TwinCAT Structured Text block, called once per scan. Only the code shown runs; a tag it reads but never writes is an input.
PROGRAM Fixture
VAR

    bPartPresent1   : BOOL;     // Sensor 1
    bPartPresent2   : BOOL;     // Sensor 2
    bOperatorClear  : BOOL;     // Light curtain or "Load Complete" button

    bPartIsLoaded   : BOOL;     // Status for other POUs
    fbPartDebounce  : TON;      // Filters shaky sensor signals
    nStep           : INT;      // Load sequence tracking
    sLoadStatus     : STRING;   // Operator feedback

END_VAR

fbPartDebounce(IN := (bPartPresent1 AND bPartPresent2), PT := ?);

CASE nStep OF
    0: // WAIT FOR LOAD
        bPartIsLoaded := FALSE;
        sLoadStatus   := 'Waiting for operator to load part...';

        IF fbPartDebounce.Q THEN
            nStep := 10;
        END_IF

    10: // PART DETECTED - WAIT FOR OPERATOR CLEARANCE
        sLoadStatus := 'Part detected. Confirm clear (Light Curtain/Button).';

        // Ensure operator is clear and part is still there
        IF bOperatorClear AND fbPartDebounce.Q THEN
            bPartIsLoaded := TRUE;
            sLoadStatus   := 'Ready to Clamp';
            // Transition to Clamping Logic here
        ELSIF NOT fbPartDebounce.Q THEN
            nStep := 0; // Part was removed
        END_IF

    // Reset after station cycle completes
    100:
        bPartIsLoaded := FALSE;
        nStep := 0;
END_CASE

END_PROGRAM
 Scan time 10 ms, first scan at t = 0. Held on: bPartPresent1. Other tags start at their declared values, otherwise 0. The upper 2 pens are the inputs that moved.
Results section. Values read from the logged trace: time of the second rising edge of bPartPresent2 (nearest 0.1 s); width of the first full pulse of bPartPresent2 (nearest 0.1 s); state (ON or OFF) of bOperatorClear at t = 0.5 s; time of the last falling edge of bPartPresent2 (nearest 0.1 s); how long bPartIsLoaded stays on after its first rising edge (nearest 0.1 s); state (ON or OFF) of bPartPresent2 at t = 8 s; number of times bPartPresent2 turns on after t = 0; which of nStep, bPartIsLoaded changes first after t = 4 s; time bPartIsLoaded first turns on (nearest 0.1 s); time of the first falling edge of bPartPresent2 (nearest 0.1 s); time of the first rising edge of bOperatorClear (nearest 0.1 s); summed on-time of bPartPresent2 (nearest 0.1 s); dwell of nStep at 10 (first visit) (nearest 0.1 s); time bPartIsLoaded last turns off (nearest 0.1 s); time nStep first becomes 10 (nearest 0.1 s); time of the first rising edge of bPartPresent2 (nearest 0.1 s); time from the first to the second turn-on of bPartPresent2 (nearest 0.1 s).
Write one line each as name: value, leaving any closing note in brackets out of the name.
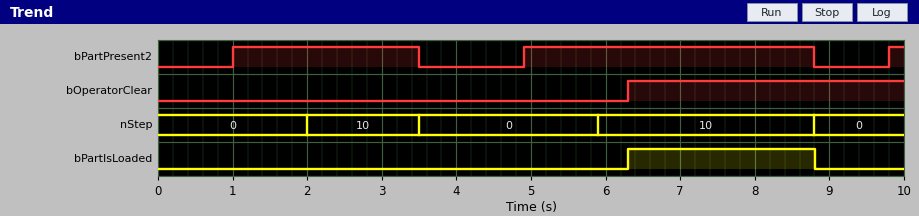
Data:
time of the second rising edge of bPartPresent2: 4.9 s
width of the first full pulse of bPartPresent2: 2.5 s
state (ON or OFF) of bOperatorClear at t = 0.5 s: OFF
time of the last falling edge of bPartPresent2: 8.8 s
how long bPartIsLoaded stays on after its first rising edge: 2.5 s
state (ON or OFF) of bPartPresent2 at t = 8 s: ON
number of times bPartPresent2 turns on after t = 0: 3
which of nStep, bPartIsLoaded changes first after t = 4 s: nStep
time bPartIsLoaded first turns on: 6.3 s
time of the first falling edge of bPartPresent2: 3.5 s
time of the first rising edge of bOperatorClear: 6.3 s
summed on-time of bPartPresent2: 6.6 s
dwell of nStep at 10 (first visit): 1.5 s
time bPartIsLoaded last turns off: 8.8 s
time nStep first becomes 10: 2.0 s
time of the first rising edge of bPartPresent2: 1.0 s
time from the first to the second turn-on of bPartPresent2: 3.9 s
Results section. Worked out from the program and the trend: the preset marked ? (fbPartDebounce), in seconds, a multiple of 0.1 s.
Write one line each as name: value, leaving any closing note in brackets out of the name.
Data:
the preset marked ? (fbPartDebounce), in seconds, a multiple of 0.1 s: 1.0 s
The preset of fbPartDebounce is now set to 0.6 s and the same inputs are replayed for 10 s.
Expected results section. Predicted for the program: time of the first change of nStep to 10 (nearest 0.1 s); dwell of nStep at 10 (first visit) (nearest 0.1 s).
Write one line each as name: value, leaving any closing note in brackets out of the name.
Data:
time of the first change of nStep to 10: 1.6 s
dwell of nStep at 10 (first visit): 1.9 s
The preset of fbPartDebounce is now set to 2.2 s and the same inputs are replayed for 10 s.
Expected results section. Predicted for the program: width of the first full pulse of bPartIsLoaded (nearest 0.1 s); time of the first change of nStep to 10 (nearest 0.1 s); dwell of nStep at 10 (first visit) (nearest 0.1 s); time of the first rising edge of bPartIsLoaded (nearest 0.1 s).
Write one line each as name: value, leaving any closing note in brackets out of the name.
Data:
width of the first full pulse of bPartIsLoaded: 1.7 s
time of the first change of nStep to 10: 3.2 s
dwell of nStep at 10 (first visit): 0.3 s
time of the first rising edge of bPartIsLoaded: 7.1 s
